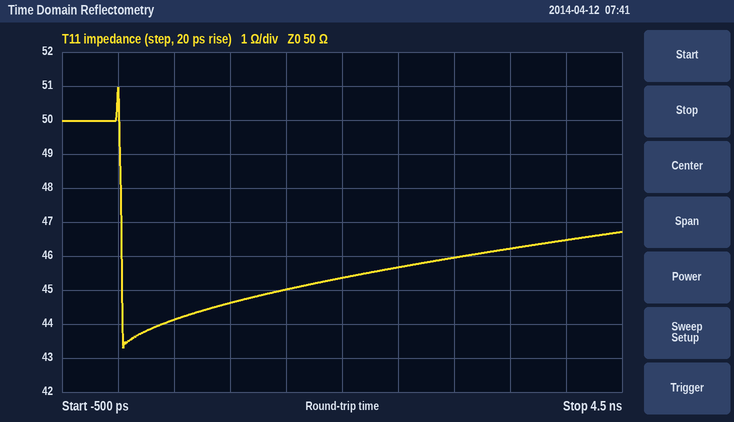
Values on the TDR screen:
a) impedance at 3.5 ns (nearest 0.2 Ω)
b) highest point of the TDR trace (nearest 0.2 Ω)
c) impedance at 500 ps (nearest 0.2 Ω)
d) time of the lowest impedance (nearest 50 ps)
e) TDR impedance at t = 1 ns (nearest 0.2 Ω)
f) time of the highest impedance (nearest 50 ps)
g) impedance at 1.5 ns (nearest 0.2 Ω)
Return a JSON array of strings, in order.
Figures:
["46.2 Ω", "51.0 Ω", "44.2 Ω", "50 ps", "44.6 Ω", "0 ps", "45.0 Ω"]
